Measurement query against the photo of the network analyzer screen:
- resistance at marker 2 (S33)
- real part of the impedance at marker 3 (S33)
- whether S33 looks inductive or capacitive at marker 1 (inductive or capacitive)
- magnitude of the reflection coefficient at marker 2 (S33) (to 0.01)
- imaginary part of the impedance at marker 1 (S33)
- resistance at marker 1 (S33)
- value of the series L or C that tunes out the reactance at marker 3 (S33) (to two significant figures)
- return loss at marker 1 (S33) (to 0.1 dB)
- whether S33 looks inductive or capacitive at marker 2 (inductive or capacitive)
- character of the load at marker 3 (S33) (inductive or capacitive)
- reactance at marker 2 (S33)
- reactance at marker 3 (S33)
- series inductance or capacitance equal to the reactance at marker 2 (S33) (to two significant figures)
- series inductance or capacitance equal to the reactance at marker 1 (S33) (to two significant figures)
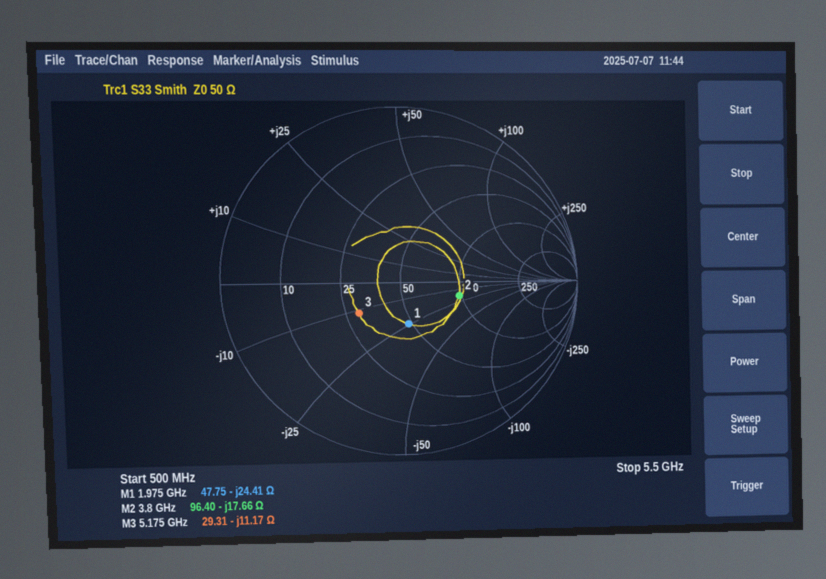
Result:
96.40 Ω
29.31 Ω
capacitive
0.34
-24.41 Ω
47.75 Ω
340 pH
12.3 dB
capacitive
capacitive
-17.66 Ω
-11.17 Ω
2.4 pF
3.3 pF
